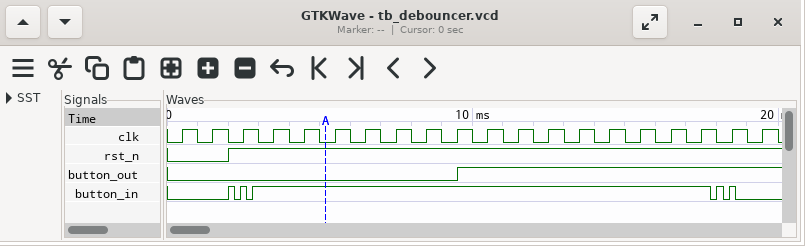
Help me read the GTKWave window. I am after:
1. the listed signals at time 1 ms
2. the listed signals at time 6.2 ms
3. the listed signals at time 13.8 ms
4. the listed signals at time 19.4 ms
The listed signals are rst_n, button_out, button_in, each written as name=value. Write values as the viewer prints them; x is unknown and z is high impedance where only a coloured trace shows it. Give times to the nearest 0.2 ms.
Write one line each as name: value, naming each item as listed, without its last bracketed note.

the listed signals at time 1 ms: rst_n=0, button_out=0, button_in=0
the listed signals at time 6.2 ms: rst_n=1, button_out=0, button_in=1
the listed signals at time 13.8 ms: rst_n=1, button_out=1, button_in=1
the listed signals at time 19.4 ms: rst_n=1, button_out=1, button_in=0
